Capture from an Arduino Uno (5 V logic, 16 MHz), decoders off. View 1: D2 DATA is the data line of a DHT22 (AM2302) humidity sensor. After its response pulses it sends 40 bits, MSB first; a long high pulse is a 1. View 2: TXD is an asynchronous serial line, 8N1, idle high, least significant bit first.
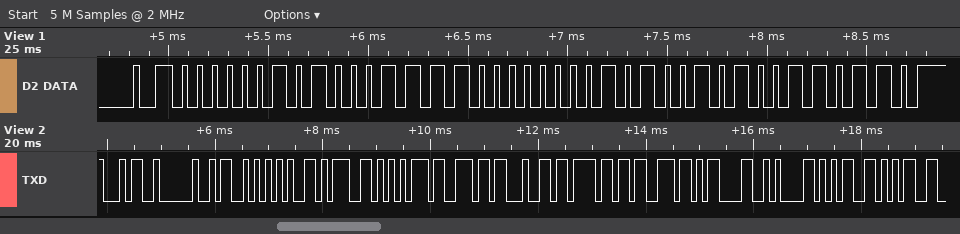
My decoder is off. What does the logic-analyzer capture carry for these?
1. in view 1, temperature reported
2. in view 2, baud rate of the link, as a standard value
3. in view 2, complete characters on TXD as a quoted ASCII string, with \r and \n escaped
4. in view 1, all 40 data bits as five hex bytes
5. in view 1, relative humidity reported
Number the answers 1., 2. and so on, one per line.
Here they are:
1. 16.5 °C
2. 9600 baud
3. "4 Segundos\r\n55"
4. 02 8F 00 A5 36
5. 65.5 %
